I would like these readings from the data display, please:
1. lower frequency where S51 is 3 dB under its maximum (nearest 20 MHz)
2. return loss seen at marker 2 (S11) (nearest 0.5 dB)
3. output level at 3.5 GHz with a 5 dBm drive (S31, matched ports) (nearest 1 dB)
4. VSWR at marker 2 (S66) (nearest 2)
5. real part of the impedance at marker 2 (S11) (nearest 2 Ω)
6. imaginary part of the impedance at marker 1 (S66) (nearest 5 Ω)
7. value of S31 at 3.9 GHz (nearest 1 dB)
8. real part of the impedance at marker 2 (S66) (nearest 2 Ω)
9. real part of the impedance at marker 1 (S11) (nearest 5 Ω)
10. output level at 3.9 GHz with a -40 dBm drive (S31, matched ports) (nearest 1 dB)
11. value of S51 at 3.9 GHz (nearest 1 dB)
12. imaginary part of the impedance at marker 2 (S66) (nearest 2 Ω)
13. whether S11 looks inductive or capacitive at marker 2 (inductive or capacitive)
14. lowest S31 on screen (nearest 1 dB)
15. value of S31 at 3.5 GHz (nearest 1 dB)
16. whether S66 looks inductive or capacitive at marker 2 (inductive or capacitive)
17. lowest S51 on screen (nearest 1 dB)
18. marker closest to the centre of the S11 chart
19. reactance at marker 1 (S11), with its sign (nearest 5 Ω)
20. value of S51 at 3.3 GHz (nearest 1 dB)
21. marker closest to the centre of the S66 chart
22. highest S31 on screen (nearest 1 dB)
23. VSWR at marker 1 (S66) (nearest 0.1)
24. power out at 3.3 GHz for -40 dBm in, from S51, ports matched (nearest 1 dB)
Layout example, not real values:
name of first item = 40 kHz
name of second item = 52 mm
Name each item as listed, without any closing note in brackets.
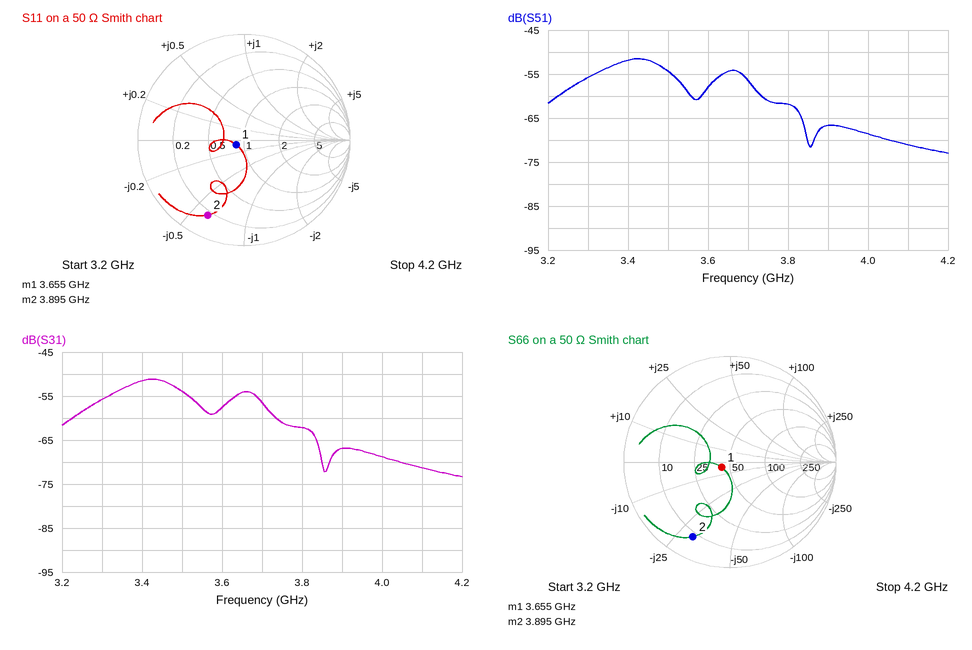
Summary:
lower frequency where S51 is 3 dB under its maximum = 3.32 GHz
return loss seen at marker 2 (S11) = 2.0 dB
output level at 3.5 GHz with a 5 dBm drive (S31, matched ports) = -49 dBm
VSWR at marker 2 (S66) = 8
real part of the impedance at marker 2 (S11) = 8 Ω
imaginary part of the impedance at marker 1 (S66) = -5 Ω
value of S31 at 3.9 GHz = -67 dB
real part of the impedance at marker 2 (S66) = 8 Ω
real part of the impedance at marker 1 (S11) = 45 Ω
output level at 3.9 GHz with a -40 dBm drive (S31, matched ports) = -107 dBm
value of S51 at 3.9 GHz = -67 dB
imaginary part of the impedance at marker 2 (S66) = -30 Ω
whether S11 looks inductive or capacitive at marker 2 = capacitive
lowest S31 on screen = -73 dB
value of S31 at 3.5 GHz = -54 dB
whether S66 looks inductive or capacitive at marker 2 = capacitive
lowest S51 on screen = -73 dB
marker closest to the centre of the S11 chart = marker 1
reactance at marker 1 (S11), with its sign = -5 Ω
value of S51 at 3.3 GHz = -56 dB
marker closest to the centre of the S66 chart = marker 1
highest S31 on screen = -51 dB
VSWR at marker 1 (S66) = 1.2
power out at 3.3 GHz for -40 dBm in, from S51, ports matched = -96 dBm
